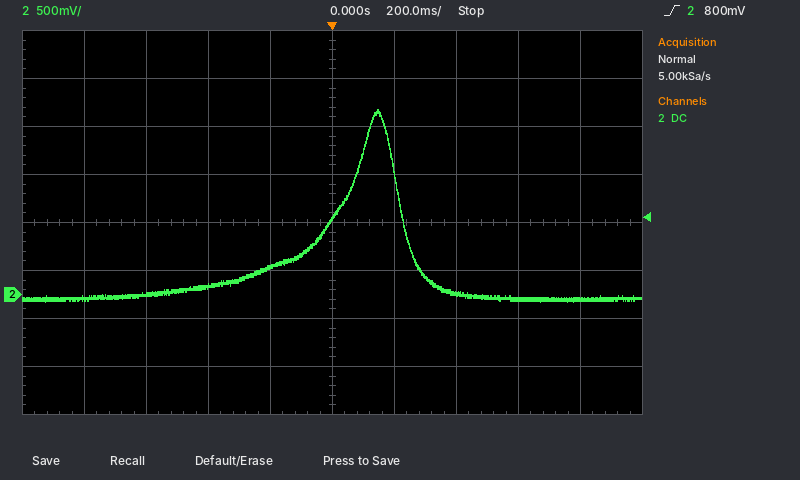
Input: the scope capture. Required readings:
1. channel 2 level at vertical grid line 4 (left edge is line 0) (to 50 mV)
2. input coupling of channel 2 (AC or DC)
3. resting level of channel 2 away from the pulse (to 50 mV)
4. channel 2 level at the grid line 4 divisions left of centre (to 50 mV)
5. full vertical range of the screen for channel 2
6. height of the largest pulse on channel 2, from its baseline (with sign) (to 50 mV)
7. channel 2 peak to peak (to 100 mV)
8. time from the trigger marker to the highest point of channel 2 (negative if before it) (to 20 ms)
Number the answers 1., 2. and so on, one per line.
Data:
1. 300 mV
2. DC
3. -50 mV
4. -50 mV
5. 4 V
6. +1.95 V
7. 2.00 V
8. +140 ms
